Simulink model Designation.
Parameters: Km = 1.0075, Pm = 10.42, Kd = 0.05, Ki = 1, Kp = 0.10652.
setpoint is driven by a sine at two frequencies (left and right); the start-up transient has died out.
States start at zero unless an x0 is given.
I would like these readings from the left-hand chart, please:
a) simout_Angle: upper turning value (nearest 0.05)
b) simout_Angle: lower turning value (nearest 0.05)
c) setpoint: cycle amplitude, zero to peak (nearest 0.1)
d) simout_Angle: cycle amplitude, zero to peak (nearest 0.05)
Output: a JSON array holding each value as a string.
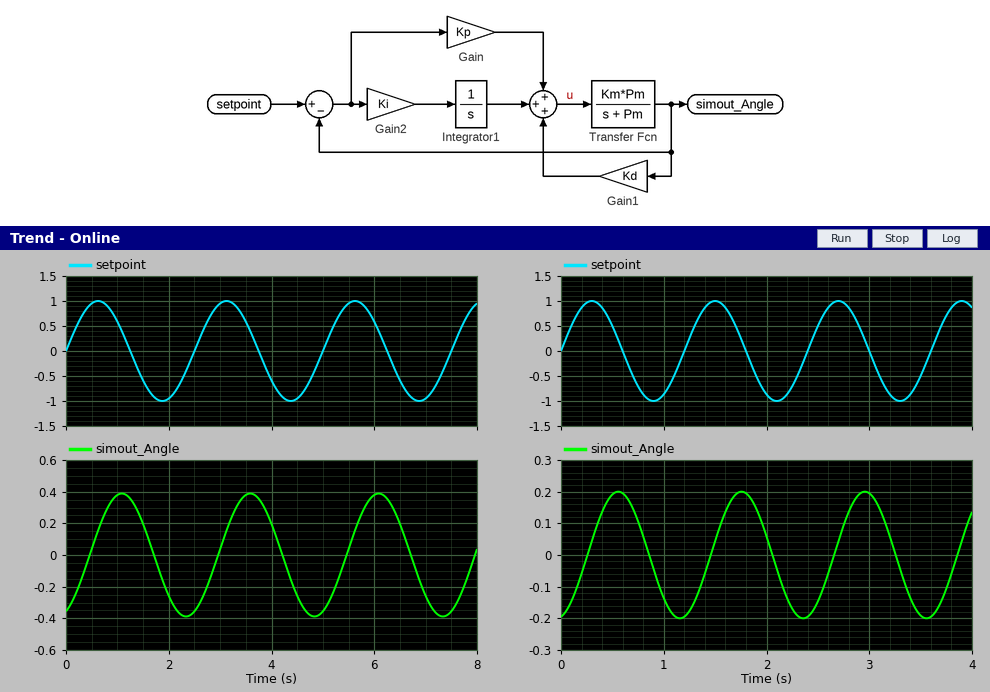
["0.40", "-0.40", "1.0", "0.40"]
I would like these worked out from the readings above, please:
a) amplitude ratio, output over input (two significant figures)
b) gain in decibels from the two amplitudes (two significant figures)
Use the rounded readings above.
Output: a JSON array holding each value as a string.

["0.40", "-8.0 dB"]
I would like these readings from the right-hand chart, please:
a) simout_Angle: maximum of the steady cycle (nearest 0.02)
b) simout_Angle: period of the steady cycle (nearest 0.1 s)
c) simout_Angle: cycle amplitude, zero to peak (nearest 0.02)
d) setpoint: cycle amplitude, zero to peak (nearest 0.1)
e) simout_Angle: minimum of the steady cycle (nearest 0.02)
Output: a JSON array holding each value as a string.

["0.20", "1.2 s", "0.20", "1.0", "-0.20"]
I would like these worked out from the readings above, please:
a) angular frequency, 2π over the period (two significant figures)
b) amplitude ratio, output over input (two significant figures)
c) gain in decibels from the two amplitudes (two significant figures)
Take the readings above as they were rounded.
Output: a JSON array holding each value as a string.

["5.2 rad/s", "0.20", "-14 dB"]
